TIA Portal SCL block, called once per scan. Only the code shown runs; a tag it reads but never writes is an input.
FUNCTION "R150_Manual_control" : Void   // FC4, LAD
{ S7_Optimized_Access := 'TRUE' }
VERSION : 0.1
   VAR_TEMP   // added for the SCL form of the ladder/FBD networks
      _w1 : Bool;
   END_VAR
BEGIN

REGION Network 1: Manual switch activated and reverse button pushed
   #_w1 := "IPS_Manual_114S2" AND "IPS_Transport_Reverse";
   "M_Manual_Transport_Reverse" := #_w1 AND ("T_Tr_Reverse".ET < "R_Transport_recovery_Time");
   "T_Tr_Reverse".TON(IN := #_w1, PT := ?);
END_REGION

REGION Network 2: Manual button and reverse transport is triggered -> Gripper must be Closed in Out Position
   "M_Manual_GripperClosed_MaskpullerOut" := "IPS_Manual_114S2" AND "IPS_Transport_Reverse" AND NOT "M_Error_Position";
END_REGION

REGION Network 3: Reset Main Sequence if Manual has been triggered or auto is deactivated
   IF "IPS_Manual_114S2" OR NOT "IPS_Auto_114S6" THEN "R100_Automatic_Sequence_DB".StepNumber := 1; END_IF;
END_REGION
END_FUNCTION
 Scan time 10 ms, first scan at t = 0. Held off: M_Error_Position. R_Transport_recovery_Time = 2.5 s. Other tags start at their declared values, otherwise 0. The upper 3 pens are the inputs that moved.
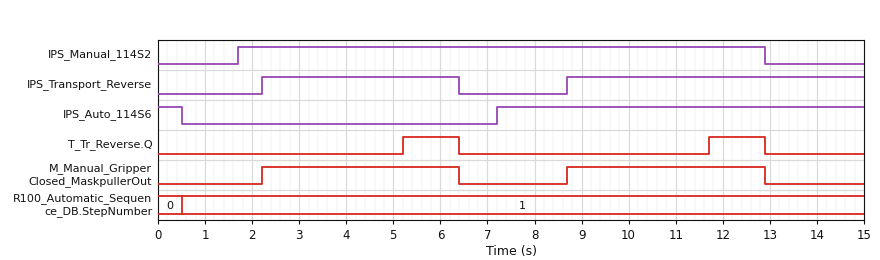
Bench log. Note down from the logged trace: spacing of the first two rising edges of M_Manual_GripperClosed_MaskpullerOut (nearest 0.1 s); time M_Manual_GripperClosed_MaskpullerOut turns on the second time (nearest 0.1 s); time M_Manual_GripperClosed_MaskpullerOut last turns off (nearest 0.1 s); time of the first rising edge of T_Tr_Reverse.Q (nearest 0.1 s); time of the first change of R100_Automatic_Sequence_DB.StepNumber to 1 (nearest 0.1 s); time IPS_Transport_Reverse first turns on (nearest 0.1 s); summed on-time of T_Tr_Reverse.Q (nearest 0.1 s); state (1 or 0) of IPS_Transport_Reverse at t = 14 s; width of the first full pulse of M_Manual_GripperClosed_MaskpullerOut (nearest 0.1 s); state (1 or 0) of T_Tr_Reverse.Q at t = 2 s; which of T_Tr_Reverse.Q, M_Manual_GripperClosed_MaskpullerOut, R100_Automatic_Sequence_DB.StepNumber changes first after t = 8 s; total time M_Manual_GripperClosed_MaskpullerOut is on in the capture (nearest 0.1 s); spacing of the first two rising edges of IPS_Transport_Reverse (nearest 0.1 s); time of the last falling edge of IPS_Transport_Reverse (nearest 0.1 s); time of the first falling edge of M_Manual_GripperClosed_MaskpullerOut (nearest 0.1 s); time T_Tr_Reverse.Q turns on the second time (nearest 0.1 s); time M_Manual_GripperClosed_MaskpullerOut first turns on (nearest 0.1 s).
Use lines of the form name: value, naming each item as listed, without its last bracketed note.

spacing of the first two rising edges of M_Manual_GripperClosed_MaskpullerOut: 6.5 s
time M_Manual_GripperClosed_MaskpullerOut turns on the second time: 8.7 s
time M_Manual_GripperClosed_MaskpullerOut last turns off: 12.9 s
time of the first rising edge of T_Tr_Reverse.Q: 5.2 s
time of the first change of R100_Automatic_Sequence_DB.StepNumber to 1: 0.5 s
time IPS_Transport_Reverse first turns on: 2.2 s
summed on-time of T_Tr_Reverse.Q: 2.4 s
state (1 or 0) of IPS_Transport_Reverse at t = 14 s: 1
width of the first full pulse of M_Manual_GripperClosed_MaskpullerOut: 4.2 s
state (1 or 0) of T_Tr_Reverse.Q at t = 2 s: 0
which of T_Tr_Reverse.Q, M_Manual_GripperClosed_MaskpullerOut, R100_Automatic_Sequence_DB.StepNumber changes first after t = 8 s: M_Manual_GripperClosed_MaskpullerOut
total time M_Manual_GripperClosed_MaskpullerOut is on in the capture: 8.4 s
spacing of the first two rising edges of IPS_Transport_Reverse: 6.5 s
time of the last falling edge of IPS_Transport_Reverse: 6.4 s
time of the first falling edge of M_Manual_GripperClosed_MaskpullerOut: 6.4 s
time T_Tr_Reverse.Q turns on the second time: 11.7 s
time M_Manual_GripperClosed_MaskpullerOut first turns on: 2.2 s
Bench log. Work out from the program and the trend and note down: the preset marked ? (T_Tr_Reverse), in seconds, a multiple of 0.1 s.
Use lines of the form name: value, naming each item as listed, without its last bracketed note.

the preset marked ? (T_Tr_Reverse), in seconds, a multiple of 0.1 s: 3.0 s
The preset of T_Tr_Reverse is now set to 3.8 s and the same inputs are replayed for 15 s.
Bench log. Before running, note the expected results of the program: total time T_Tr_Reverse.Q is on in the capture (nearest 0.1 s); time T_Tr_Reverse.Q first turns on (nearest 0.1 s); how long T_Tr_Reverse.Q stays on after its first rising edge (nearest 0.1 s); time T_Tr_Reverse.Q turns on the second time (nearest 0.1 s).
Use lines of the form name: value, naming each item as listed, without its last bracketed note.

total time T_Tr_Reverse.Q is on in the capture: 0.8 s
time T_Tr_Reverse.Q first turns on: 6.0 s
how long T_Tr_Reverse.Q stays on after its first rising edge: 0.4 s
time T_Tr_Reverse.Q turns on the second time: 12.5 s
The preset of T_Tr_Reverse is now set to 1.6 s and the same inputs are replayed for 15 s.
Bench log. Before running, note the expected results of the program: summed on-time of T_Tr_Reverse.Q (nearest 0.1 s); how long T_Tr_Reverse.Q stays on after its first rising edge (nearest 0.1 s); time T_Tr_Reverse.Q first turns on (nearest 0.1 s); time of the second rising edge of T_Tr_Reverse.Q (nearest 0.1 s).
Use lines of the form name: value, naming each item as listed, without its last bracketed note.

summed on-time of T_Tr_Reverse.Q: 5.2 s
how long T_Tr_Reverse.Q stays on after its first rising edge: 2.6 s
time T_Tr_Reverse.Q first turns on: 3.8 s
time of the second rising edge of T_Tr_Reverse.Q: 10.3 s
